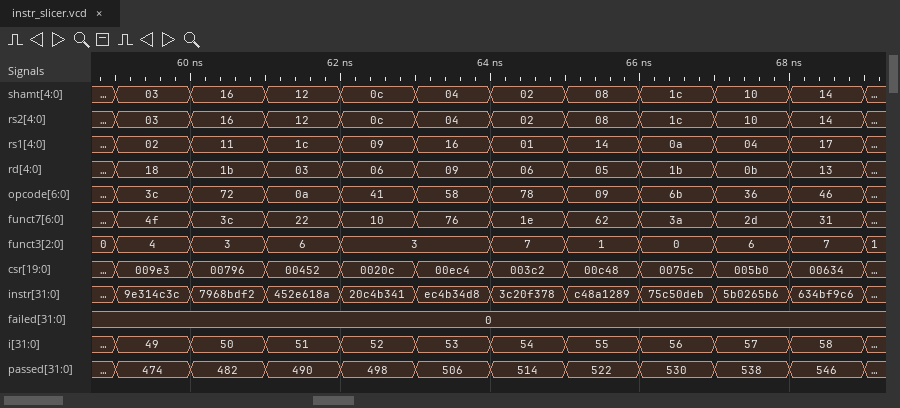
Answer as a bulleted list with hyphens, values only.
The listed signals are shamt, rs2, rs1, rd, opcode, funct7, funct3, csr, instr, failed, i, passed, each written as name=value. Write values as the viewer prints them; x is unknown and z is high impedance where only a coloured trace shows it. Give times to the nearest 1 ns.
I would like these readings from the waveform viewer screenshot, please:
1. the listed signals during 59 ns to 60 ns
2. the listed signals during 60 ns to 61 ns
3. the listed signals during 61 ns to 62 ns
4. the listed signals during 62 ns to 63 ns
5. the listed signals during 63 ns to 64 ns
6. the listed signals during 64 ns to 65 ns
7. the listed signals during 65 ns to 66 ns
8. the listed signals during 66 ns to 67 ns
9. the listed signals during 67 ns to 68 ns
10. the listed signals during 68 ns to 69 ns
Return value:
- shamt=03, rs2=03, rs1=02, rd=18, opcode=3c, funct7=4f, funct3=4, csr=009e3, instr=9e314c3c, failed=0, i=49, passed=474
- shamt=16, rs2=16, rs1=11, rd=1b, opcode=72, funct7=3c, funct3=3, csr=00796, instr=7968bdf2, failed=0, i=50, passed=482
- shamt=12, rs2=12, rs1=1c, rd=03, opcode=0a, funct7=22, funct3=6, csr=00452, instr=452e618a, failed=0, i=51, passed=490
- shamt=0c, rs2=0c, rs1=09, rd=06, opcode=41, funct7=10, funct3=3, csr=0020c, instr=20c4b341, failed=0, i=52, passed=498
- shamt=04, rs2=04, rs1=16, rd=09, opcode=58, funct7=76, funct3=3, csr=00ec4, instr=ec4b34d8, failed=0, i=53, passed=506
- shamt=02, rs2=02, rs1=01, rd=06, opcode=78, funct7=1e, funct3=7, csr=003c2, instr=3c20f378, failed=0, i=54, passed=514
- shamt=08, rs2=08, rs1=14, rd=05, opcode=09, funct7=62, funct3=1, csr=00c48, instr=c48a1289, failed=0, i=55, passed=522
- shamt=1c, rs2=1c, rs1=0a, rd=1b, opcode=6b, funct7=3a, funct3=0, csr=0075c, instr=75c50deb, failed=0, i=56, passed=530
- shamt=10, rs2=10, rs1=04, rd=0b, opcode=36, funct7=2d, funct3=6, csr=005b0, instr=5b0265b6, failed=0, i=57, passed=538
- shamt=14, rs2=14, rs1=17, rd=13, opcode=46, funct7=31, funct3=7, csr=00634, instr=634bf9c6, failed=0, i=58, passed=546
